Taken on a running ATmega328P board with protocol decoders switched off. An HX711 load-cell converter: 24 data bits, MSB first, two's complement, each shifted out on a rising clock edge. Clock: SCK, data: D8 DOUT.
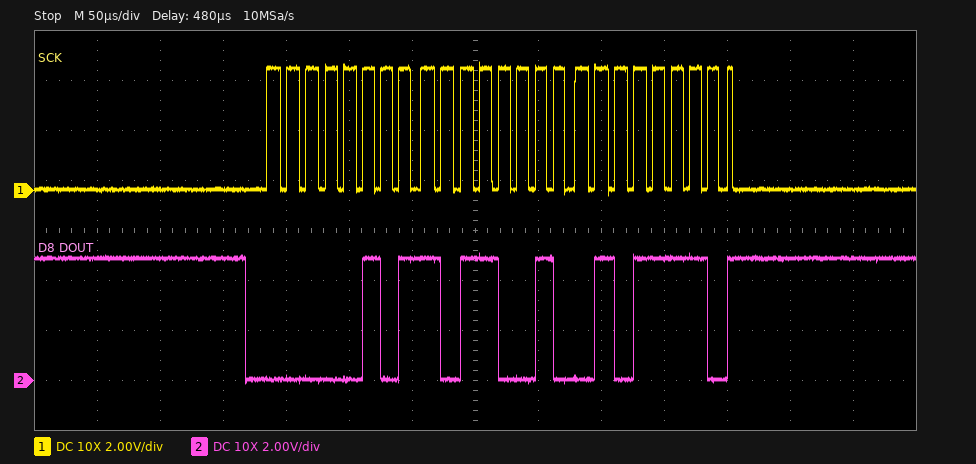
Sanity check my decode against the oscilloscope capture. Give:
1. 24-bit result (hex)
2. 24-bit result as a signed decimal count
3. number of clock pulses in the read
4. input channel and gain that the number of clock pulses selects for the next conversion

0x05B25E
373342
25
channel A, gain 128
